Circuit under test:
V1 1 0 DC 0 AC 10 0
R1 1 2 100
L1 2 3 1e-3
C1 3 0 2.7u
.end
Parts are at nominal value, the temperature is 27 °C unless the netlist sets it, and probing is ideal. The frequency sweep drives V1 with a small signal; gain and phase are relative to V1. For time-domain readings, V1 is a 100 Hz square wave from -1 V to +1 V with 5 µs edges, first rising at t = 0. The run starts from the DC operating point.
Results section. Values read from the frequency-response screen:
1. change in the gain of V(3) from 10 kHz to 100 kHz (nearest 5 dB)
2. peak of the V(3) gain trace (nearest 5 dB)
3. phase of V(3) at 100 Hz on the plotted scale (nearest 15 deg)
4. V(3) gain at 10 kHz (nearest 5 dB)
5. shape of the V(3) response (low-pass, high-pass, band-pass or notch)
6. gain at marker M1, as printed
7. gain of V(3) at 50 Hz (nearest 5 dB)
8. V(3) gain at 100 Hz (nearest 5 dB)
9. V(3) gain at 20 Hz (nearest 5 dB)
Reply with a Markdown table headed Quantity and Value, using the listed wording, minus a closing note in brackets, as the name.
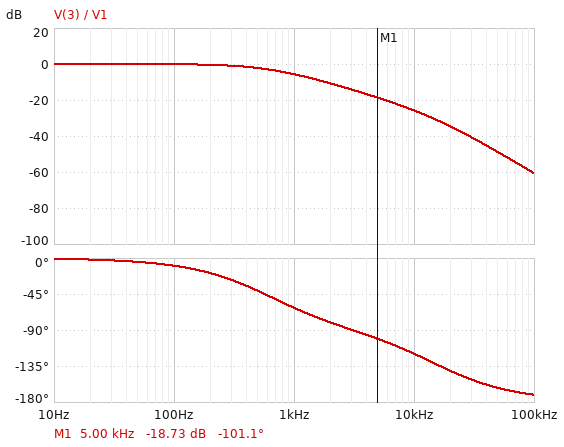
| Quantity | Value |
|---|---|
| change in the gain of V(3) from 10 kHz to 100 kHz | -35 dB |
| peak of the V(3) gain trace | 0 dB |
| phase of V(3) at 100 Hz on the plotted scale | -15 deg |
| V(3) gain at 10 kHz | -25 dB |
| shape of the V(3) response | low-pass |
| gain at marker M1, as printed | -18.73 dB |
| gain of V(3) at 50 Hz | 0 dB |
| V(3) gain at 100 Hz | 0 dB |
| V(3) gain at 20 Hz | 0 dB |
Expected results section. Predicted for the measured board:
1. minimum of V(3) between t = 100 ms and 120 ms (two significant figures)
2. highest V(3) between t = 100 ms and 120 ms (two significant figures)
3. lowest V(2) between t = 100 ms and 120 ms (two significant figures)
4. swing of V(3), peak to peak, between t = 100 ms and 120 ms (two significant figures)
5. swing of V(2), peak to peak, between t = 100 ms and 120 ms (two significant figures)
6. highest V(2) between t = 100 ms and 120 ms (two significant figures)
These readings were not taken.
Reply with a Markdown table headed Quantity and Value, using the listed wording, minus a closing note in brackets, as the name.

| Quantity | Value |
|---|---|
| minimum of V(3) between t = 100 ms and 120 ms | -1.0 V |
| highest V(3) between t = 100 ms and 120 ms | 1.0 V |
| lowest V(2) between t = 100 ms and 120 ms | -1.0 V |
| swing of V(3), peak to peak, between t = 100 ms and 120 ms | 2.0 V |
| swing of V(2), peak to peak, between t = 100 ms and 120 ms | 2.0 V |
| highest V(2) between t = 100 ms and 120 ms | 1.0 V |
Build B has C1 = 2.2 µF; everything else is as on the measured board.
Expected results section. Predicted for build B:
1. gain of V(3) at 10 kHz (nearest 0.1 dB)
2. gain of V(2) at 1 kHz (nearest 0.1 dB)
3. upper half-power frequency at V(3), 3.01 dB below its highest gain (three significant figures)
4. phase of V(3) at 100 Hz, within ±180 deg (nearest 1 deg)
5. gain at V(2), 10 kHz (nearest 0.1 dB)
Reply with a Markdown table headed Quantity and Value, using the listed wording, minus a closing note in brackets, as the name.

| Quantity | Value |
|---|---|
| gain of V(3) at 10 kHz | -24.0 dB |
| gain of V(2) at 1 kHz | -5.2 dB |
| upper half-power frequency at V(3), 3.01 dB below its highest gain | 758 Hz |
| phase of V(3) at 100 Hz, within ±180 deg | -8 deg |
| gain at V(2), 10 kHz | -6.3 dB |
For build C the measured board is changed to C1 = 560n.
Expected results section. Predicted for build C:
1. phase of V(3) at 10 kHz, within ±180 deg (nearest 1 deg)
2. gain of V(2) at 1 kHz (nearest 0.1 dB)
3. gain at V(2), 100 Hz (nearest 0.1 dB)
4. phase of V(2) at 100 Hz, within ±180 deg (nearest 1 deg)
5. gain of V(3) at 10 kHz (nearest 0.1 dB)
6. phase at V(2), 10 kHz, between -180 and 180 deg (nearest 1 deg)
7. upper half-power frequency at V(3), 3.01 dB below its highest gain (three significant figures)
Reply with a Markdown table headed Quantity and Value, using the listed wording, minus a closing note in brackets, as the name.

| Quantity | Value |
|---|---|
| phase of V(3) at 10 kHz, within ±180 deg | -109 deg |
| gain of V(2) at 1 kHz | -0.5 dB |
| gain at V(2), 100 Hz | 0 dB |
| phase of V(2) at 100 Hz, within ±180 deg | -2 deg |
| gain of V(3) at 10 kHz | -11.4 dB |
| phase at V(2), 10 kHz, between -180 and 180 deg | 71 deg |
| upper half-power frequency at V(3), 3.01 dB below its highest gain | 3.42 kHz |
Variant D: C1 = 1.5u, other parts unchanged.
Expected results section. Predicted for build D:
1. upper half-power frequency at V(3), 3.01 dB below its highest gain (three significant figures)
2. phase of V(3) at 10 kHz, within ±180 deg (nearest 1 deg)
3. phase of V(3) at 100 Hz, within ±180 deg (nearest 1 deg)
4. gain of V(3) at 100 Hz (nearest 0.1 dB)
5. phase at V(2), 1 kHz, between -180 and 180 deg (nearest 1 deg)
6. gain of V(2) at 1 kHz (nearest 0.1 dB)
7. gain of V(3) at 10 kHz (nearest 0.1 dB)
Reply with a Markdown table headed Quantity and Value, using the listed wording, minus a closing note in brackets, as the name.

| Quantity | Value |
|---|---|
| upper half-power frequency at V(3), 3.01 dB below its highest gain | 1.14 kHz |
| phase of V(3) at 10 kHz, within ±180 deg | -118 deg |
| phase of V(3) at 100 Hz, within ±180 deg | -5 deg |
| gain of V(3) at 100 Hz | 0 dB |
| phase at V(2), 1 kHz, between -180 and 180 deg | -45 deg |
| gain of V(2) at 1 kHz | -3.0 dB |
| gain of V(3) at 10 kHz | -20.5 dB |
